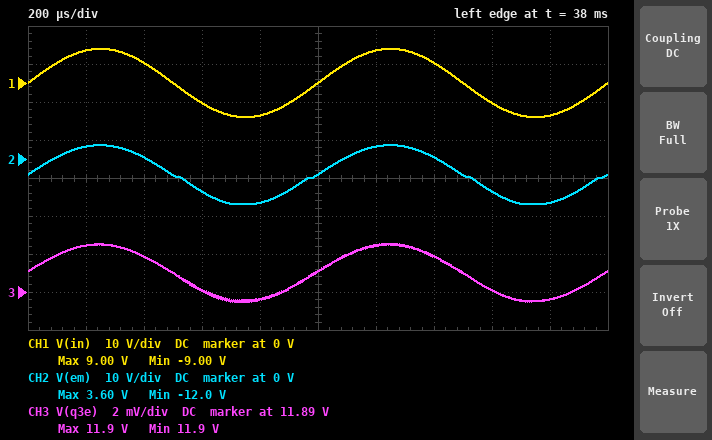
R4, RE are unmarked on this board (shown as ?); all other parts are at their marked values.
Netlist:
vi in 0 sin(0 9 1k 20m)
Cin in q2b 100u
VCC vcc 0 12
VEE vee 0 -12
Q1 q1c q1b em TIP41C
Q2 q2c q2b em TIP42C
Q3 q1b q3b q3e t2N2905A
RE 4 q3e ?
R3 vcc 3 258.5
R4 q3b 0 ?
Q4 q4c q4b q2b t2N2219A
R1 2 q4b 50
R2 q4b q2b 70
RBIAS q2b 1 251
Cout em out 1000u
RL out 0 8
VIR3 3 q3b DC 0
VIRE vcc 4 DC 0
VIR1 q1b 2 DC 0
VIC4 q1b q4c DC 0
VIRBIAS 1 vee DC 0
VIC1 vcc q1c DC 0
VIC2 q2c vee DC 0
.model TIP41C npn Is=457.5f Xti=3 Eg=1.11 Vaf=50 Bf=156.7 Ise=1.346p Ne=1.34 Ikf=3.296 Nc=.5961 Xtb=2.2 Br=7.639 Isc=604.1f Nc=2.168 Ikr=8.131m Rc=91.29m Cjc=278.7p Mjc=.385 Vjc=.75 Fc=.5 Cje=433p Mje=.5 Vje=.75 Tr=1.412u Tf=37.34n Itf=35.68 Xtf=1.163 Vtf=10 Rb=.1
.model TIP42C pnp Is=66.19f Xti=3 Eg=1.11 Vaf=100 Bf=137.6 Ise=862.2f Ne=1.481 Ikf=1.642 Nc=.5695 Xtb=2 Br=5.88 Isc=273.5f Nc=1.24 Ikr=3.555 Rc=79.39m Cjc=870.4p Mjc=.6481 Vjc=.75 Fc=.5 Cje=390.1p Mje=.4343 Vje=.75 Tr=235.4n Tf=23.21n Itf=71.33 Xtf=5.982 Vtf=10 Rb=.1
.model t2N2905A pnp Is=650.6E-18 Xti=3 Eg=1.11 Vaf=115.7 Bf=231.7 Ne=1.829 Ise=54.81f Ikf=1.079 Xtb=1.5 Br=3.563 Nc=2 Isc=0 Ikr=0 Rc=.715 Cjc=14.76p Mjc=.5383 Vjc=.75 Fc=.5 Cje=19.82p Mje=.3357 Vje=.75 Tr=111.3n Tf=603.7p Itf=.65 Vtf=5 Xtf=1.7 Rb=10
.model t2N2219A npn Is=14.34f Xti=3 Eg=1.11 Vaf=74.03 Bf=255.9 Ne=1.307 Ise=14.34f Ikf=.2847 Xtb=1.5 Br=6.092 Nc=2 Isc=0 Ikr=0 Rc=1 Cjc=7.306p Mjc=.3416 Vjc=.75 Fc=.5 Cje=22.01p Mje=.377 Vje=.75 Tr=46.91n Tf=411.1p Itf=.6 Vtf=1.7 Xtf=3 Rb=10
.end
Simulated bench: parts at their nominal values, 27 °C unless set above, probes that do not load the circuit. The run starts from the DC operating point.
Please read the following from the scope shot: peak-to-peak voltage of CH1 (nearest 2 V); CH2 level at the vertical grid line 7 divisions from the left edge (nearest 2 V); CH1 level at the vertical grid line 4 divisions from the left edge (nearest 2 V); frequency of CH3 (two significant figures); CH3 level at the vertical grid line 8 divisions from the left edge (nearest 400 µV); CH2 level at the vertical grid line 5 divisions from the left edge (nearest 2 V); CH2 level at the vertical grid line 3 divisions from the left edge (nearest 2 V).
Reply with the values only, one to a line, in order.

18 V
0 V
-8 V
1.0 kHz
11.8900 V
-4 V
-8 V
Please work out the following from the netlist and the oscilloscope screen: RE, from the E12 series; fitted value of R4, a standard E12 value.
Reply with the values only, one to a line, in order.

27 Ω
3.3 kΩ
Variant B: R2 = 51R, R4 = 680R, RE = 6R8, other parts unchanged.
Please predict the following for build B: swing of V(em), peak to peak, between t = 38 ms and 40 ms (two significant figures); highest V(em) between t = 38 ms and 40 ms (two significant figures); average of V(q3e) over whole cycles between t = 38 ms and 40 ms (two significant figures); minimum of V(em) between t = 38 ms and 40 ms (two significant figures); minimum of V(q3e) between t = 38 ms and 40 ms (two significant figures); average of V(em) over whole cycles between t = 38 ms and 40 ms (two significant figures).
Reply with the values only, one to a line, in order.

10 V
12 V
11 V
1.7 V
9.9 V
8.3 V
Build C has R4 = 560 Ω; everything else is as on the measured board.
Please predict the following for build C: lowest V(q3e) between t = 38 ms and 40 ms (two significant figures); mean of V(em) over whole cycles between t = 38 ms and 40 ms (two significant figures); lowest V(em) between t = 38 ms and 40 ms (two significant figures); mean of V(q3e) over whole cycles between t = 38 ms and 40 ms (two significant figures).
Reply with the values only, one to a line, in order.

9.1 V
5.2 V
-2.9 V
10 V
